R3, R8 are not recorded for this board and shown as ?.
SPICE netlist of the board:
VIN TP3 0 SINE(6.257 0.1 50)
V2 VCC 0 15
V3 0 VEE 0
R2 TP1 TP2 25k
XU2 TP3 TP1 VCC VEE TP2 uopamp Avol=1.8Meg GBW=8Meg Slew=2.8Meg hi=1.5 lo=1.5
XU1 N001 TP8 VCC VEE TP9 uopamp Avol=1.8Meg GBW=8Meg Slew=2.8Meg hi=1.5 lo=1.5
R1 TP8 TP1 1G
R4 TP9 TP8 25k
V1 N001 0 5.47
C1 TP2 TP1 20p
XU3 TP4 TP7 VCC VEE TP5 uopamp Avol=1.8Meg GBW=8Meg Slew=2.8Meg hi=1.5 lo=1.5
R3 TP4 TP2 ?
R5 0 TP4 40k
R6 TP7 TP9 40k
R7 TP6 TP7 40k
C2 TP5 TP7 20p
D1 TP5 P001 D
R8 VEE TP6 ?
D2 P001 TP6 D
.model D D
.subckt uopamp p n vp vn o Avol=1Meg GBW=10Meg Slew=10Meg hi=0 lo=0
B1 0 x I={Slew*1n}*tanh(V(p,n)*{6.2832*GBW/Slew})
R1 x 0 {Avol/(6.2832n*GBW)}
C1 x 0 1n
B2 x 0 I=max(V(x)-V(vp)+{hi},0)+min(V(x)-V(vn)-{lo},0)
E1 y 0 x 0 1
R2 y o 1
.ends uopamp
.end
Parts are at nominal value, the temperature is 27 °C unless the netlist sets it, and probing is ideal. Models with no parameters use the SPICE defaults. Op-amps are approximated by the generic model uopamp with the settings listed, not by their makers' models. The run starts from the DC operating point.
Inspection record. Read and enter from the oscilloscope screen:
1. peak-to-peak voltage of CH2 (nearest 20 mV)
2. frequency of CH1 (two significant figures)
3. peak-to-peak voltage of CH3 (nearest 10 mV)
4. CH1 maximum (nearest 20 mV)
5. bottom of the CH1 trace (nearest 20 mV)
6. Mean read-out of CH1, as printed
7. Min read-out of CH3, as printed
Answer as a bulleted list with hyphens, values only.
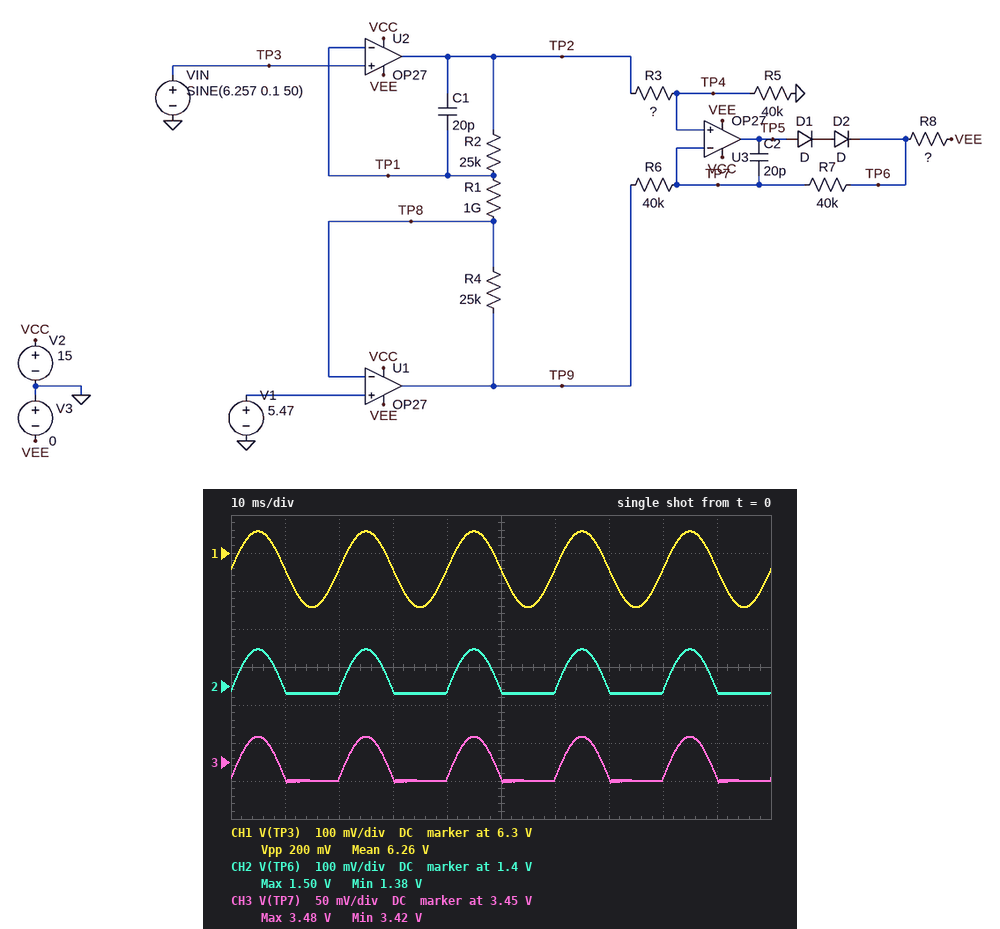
- 120 mV
- 50 Hz
- 60 mV
- 6.36 V
- 6.16 V
- 6.26 V
- 3.42 V
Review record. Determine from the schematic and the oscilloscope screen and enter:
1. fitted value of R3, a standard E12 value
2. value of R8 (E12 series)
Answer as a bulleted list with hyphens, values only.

- 33 kΩ
- 27 kΩ
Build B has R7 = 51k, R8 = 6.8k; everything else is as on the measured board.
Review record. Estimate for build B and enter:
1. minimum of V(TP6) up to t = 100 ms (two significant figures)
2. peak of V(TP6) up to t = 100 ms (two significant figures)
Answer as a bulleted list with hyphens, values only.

- 700 mV
- 950 mV
